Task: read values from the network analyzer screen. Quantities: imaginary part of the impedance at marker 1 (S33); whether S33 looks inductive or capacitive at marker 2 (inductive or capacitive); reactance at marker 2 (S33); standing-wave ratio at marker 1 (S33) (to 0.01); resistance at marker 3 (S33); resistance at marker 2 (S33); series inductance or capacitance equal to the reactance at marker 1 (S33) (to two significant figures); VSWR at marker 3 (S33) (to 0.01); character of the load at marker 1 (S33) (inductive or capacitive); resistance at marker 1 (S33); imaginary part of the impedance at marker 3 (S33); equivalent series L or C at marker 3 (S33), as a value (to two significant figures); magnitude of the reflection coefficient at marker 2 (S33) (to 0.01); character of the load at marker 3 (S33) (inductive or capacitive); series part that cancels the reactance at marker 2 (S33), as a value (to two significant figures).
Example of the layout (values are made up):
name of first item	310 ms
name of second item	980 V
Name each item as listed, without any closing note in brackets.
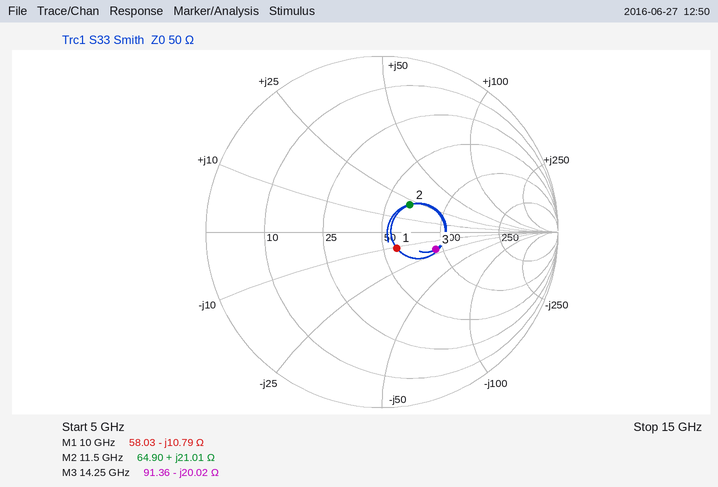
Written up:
imaginary part of the impedance at marker 1	-10.79 Ω
whether S33 looks inductive or capacitive at marker 2	inductive
reactance at marker 2	+21.01 Ω
standing-wave ratio at marker 1 (S33)	1.28
resistance at marker 3	91.36 Ω
resistance at marker 2	64.90 Ω
series inductance or capacitance equal to the reactance at marker 1 (S33)	1.5 pF
VSWR at marker 3 (S33)	1.95
character of the load at marker 1 (S33)	capacitive
resistance at marker 1	58.03 Ω
imaginary part of the impedance at marker 3	-20.02 Ω
equivalent series L or C at marker 3 (S33), as a value	560 fF
magnitude of the reflection coefficient at marker 2 (S33)	0.22
character of the load at marker 3 (S33)	capacitive
series part that cancels the reactance at marker 2 (S33), as a value	660 fF
